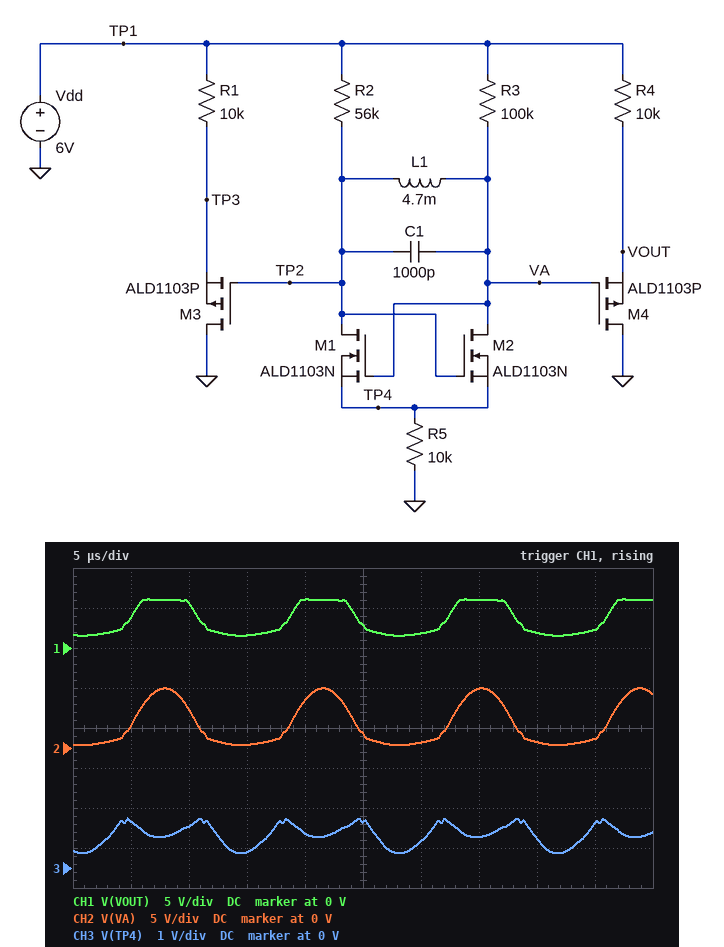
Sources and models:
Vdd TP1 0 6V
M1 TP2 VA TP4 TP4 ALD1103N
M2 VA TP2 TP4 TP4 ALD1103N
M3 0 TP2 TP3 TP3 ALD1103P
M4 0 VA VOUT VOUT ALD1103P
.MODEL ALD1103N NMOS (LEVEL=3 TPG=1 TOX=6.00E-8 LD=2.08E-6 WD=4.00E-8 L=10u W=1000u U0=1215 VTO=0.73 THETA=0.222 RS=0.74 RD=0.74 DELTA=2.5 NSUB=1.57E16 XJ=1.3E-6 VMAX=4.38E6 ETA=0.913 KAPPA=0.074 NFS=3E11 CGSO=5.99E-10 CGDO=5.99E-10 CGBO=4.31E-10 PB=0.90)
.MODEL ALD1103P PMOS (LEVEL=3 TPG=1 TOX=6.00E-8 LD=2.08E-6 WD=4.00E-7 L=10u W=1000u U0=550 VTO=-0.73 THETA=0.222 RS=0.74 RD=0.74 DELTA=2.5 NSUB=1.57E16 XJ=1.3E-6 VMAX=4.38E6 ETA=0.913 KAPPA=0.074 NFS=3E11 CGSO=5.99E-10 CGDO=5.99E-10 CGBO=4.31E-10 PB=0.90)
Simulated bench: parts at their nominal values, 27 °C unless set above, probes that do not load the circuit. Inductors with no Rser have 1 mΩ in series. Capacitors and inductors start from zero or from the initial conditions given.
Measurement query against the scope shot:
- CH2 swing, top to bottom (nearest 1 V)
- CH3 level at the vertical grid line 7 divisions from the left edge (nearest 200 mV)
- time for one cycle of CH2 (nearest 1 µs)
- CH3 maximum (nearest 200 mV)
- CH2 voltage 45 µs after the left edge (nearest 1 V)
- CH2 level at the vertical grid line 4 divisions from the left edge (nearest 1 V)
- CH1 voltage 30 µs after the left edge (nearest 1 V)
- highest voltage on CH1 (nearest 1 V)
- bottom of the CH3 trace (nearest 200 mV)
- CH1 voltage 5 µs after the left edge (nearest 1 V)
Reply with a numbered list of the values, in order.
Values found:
1. 7 V
2. 800 mV
3. 14 µs
4. 1.2 V
5. 1 V
6. 6 V
7. 2 V
8. 6 V
9. 400 mV
10. 4 V
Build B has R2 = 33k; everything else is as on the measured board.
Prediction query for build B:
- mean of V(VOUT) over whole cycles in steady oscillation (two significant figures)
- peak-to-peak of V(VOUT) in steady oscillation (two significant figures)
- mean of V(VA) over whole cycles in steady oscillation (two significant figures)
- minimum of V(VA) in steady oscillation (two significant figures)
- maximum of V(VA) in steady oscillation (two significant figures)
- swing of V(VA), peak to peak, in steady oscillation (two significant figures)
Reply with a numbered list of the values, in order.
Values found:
1. 3.7 V
2. 4.6 V
3. 3.3 V
4. 290 mV
5. 7.9 V
6. 7.6 V
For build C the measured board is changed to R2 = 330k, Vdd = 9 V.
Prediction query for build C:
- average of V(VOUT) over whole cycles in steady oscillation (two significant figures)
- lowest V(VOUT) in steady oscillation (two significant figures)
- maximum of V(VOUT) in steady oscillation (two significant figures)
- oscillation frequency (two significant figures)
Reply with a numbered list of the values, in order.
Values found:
1. 4.7 V
2. 2.0 V
3. 9.1 V
4. 73 kHz
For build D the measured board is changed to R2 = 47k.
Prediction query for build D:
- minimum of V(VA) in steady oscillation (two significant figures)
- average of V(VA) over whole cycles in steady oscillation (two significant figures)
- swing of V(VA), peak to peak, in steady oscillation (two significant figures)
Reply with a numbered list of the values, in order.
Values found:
1. 340 mV
2. 3.1 V
3. 7.3 V
